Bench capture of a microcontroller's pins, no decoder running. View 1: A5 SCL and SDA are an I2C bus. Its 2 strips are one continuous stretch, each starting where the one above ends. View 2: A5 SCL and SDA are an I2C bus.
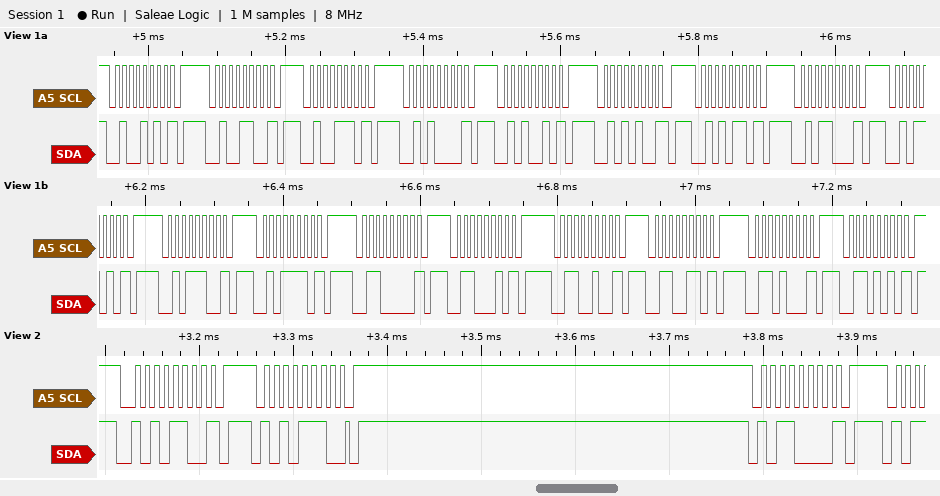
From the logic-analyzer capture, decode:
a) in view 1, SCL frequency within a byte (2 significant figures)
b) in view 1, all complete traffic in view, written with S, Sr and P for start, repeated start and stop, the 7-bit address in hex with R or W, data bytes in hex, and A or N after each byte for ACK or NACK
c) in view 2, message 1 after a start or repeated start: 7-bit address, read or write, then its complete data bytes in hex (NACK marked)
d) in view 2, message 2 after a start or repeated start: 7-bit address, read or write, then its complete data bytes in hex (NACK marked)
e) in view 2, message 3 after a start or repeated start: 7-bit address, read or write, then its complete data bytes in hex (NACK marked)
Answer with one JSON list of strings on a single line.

["100 kHz", "S 25W N P S 26W N P S 27W N P S 28W N P S 29W N P S 2AW N P S 2BW N P S 2CW N P S 2DW N P S 2EW N P S 2FW N P S 30W N P S 31W N P S 32W N P S 33W N P S 34W N P S 35W N P", "0x56 write NACK", "0x57 write", "0x58 write NACK"]
